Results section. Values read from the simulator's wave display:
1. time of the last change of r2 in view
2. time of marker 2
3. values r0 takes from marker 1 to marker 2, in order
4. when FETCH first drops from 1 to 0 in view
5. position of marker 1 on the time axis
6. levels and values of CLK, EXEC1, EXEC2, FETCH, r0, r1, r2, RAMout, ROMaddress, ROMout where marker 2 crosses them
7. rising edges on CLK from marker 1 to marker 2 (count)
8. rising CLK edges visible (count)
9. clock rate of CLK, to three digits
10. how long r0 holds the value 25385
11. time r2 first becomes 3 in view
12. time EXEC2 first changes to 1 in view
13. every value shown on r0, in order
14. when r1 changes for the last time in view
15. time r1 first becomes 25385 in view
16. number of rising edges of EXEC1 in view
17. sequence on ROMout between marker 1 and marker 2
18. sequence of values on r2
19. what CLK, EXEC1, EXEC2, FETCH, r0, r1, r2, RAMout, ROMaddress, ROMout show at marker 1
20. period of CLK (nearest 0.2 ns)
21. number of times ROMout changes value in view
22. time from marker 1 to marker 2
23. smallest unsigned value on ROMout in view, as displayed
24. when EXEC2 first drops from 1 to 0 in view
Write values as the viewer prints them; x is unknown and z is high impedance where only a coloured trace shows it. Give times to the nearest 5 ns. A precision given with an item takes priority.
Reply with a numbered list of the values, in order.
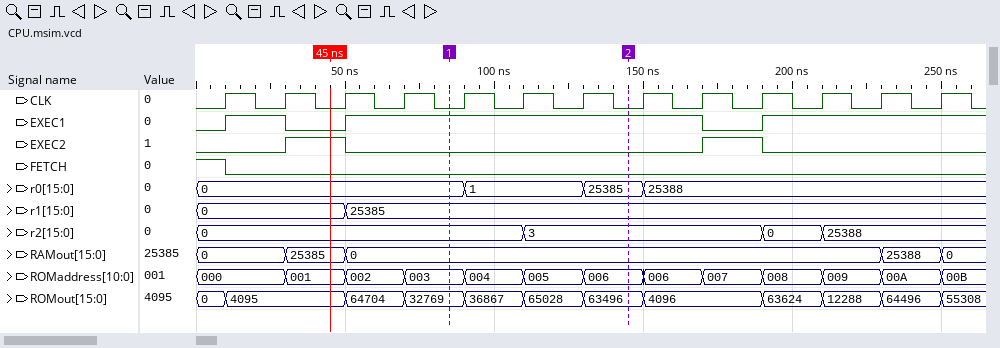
1. 210 ns
2. 145 ns
3. 0, 1, 25385
4. 10 ns
5. 85 ns
6. CLK=0, EXEC1=1, EXEC2=0, FETCH=0, r0=25385, r1=25385, r2=3, RAMout=0, ROMaddress=006, ROMout=63496
7. 3
8. 13
9. 50.0 MHz
10. 20 ns
11. 110 ns
12. 30 ns
13. 0, 1, 25385, 25388
14. 50 ns
15. 50 ns
16. 3
17. 32769, 36867, 65028, 63496
18. 0, 3, 0, 25388
19. CLK=0, EXEC1=1, EXEC2=0, FETCH=0, r0=0, r1=25385, r2=0, RAMout=0, ROMaddress=003, ROMout=32769
20. 20 ns
21. 11
22. 60 ns
23. 0
24. 50 ns
